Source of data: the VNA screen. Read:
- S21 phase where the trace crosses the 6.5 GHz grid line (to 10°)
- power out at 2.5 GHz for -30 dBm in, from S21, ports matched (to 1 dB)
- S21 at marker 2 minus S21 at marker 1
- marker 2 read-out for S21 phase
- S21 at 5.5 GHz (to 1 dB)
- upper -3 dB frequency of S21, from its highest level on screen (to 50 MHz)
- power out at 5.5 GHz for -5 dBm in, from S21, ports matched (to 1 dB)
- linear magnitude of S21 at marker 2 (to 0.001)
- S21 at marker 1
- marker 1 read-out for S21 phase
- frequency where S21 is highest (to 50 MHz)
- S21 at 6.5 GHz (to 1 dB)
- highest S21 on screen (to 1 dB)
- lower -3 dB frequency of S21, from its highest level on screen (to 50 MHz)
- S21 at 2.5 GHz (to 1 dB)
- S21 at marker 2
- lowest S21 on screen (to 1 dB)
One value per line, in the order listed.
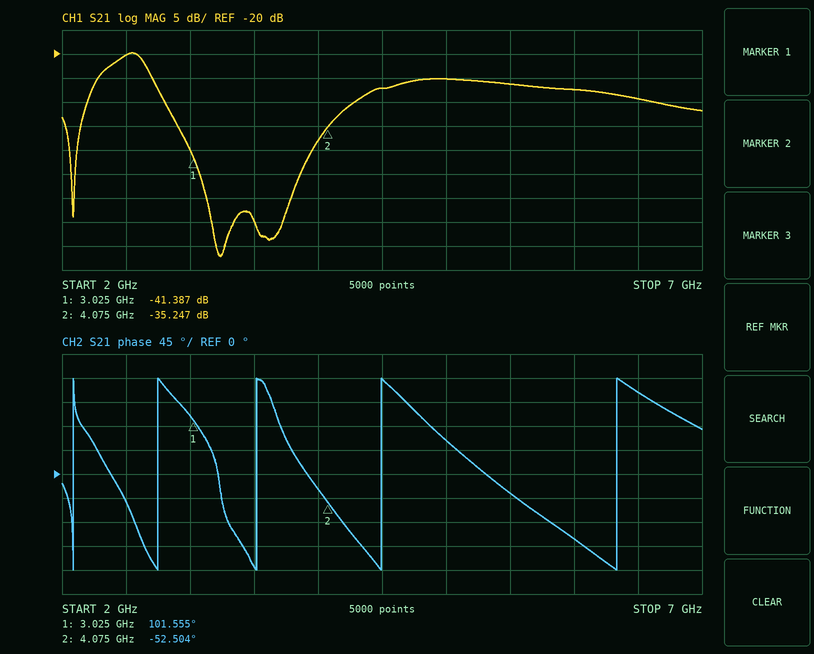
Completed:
150°
-50 dBm
6.140 dB
-52.504°
-26 dB
2.65 GHz
-31 dBm
0.017
-41.387 dB
101.555°
2.55 GHz
-29 dB
-20 dB
2.35 GHz
-20 dB
-35.247 dB
-62 dB
